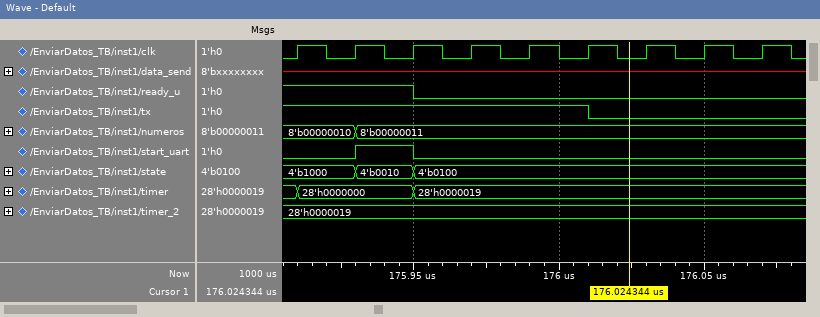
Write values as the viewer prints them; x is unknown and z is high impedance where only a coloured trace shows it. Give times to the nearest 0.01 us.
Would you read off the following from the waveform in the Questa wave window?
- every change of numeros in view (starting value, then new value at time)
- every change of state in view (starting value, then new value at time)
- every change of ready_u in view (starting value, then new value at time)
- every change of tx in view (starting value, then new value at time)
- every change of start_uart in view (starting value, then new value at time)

8'b00000010, 8'b00000011 at 175.93 us
4'b1000, 4'b0010 at 175.93 us, 4'b0100 at 175.95 us
1, 0 at 175.95 us
1, 0 at 176.01 us
0, 1 at 175.93 us, 0 at 175.95 us
